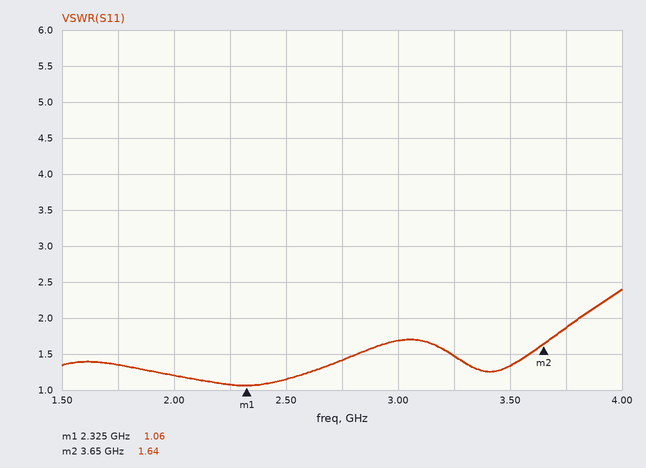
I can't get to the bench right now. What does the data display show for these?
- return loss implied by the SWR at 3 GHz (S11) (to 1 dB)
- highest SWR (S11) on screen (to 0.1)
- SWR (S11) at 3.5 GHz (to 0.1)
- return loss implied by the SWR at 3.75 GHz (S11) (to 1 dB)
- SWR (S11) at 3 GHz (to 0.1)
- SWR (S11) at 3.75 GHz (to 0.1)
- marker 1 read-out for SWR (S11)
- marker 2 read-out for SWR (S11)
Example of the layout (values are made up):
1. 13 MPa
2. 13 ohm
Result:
1. 12 dB
2. 2.4
3. 1.3
4. 10 dB
5. 1.7
6. 1.9
7. 1.06
8. 1.64
